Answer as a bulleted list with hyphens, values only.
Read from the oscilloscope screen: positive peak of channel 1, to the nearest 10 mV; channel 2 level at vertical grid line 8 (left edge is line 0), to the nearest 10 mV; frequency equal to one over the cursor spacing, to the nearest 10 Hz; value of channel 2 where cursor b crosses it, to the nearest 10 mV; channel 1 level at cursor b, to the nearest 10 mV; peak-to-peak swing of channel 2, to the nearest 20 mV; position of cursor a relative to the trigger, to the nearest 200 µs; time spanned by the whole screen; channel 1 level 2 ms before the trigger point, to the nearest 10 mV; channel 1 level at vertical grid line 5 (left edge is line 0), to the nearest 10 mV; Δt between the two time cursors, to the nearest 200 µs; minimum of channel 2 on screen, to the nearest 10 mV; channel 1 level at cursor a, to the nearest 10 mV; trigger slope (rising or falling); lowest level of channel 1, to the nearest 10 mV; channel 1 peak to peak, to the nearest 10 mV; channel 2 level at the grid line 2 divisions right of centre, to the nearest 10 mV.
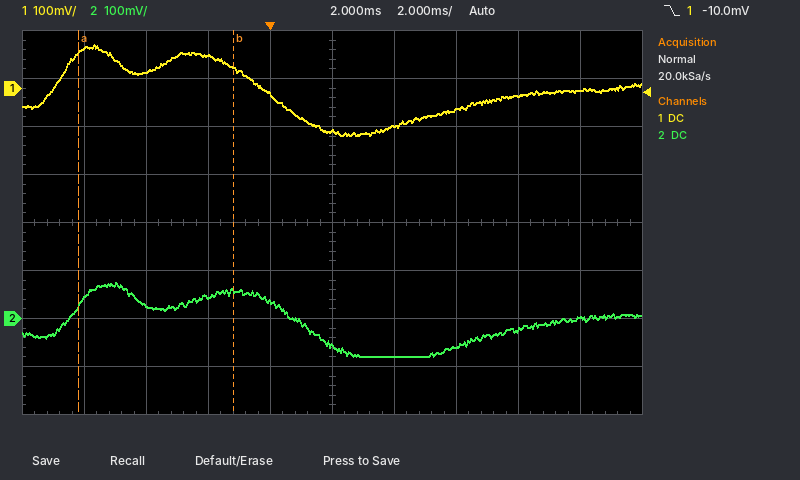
- 90 mV
- -20 mV
- 200 Hz
- 60 mV
- 40 mV
- 160 mV
- -6.2 ms
- 20 ms
- 70 mV
- -90 mV
- 5.0 ms
- -80 mV
- 70 mV
- falling
- -100 mV
- 190 mV
- -60 mV
